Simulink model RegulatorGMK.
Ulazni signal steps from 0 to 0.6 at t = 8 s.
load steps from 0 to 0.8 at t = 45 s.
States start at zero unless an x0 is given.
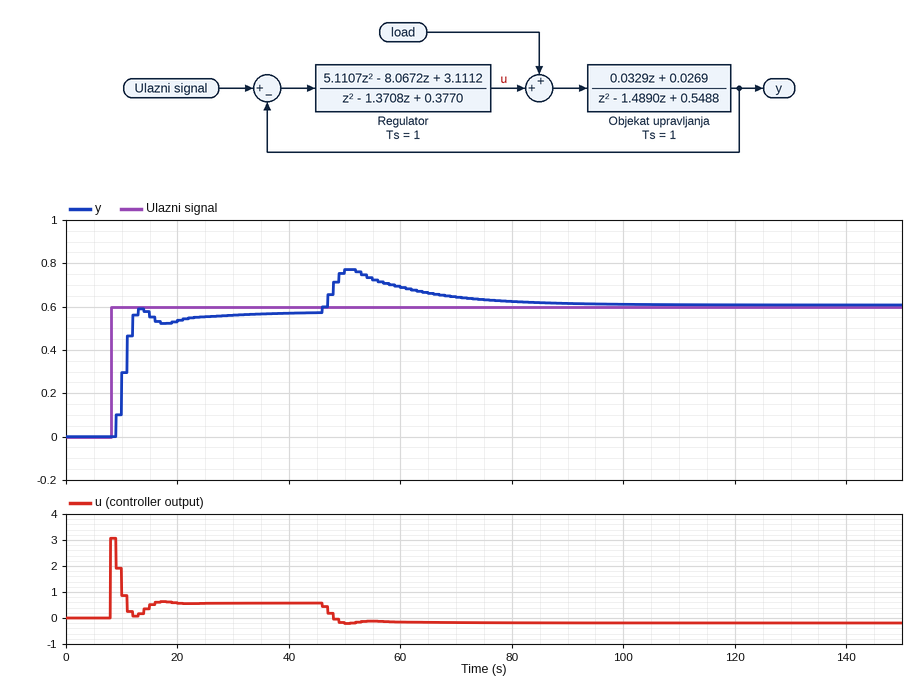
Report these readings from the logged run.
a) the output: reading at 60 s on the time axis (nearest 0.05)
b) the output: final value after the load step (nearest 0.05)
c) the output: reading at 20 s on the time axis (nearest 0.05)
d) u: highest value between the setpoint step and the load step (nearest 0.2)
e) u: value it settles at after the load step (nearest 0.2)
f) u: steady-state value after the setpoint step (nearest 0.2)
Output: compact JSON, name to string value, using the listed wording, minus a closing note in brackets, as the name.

{"the output: reading at 60 s on the time axis": "0.70", "the output: final value after the load step": "0.60", "the output: reading at 20 s on the time axis": "0.55", "u: highest value between the setpoint step and the load step": "3.0", "u: value it settles at after the load step": "-0.2", "u: steady-state value after the setpoint step": "0.6"}
